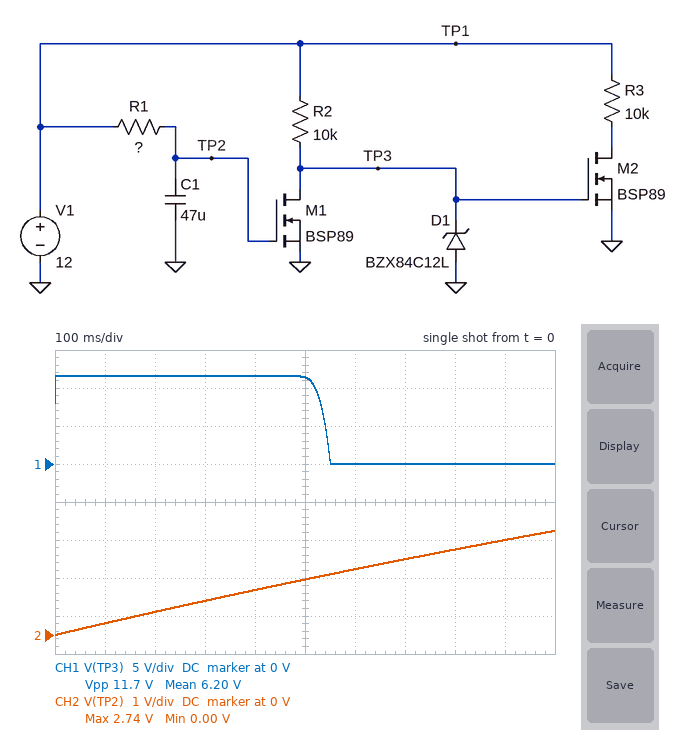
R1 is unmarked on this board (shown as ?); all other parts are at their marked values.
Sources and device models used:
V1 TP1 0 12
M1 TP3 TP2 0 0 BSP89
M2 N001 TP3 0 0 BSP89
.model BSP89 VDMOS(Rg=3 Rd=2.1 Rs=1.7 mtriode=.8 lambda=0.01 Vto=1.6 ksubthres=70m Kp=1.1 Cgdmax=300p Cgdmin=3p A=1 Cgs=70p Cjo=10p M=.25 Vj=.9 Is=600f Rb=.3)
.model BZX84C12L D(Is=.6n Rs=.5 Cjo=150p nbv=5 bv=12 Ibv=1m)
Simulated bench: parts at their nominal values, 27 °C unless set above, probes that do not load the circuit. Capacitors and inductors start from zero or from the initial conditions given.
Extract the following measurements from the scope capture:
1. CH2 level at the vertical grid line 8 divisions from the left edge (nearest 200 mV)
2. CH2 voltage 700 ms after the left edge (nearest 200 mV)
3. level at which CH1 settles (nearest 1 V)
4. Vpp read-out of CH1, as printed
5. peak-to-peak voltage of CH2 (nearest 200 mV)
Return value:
2.2 V
2.0 V
0 V
11.7 V
2.8 V
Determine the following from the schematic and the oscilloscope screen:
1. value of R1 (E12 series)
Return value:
82 kΩ
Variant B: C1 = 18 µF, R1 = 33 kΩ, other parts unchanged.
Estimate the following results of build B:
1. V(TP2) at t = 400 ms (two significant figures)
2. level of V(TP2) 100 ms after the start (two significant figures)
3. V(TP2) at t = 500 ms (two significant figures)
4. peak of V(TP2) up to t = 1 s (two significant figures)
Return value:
5.9 V
1.9 V
6.8 V
9.8 V
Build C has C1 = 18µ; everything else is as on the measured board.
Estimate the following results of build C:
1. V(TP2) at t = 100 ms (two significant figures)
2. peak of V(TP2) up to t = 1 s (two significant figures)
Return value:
790 mV
5.9 V
